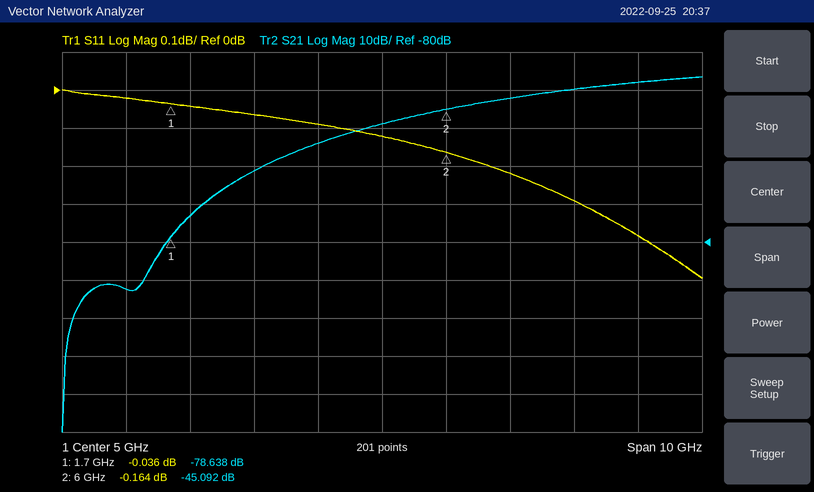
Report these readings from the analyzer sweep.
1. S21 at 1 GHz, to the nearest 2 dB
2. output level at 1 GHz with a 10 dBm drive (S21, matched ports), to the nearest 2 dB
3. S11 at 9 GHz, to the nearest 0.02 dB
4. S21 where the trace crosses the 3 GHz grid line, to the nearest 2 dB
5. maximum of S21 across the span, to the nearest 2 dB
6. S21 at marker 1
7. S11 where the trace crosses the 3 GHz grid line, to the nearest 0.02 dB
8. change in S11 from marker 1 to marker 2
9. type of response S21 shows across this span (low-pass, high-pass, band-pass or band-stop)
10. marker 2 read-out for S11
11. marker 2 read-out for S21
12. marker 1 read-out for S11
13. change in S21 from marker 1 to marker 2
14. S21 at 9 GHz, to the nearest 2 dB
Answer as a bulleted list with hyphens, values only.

- -92 dB
- -82 dBm
- -0.38 dB
- -62 dB
- -36 dB
- -78.638 dB
- -0.06 dB
- -0.128 dB
- high-pass
- -0.164 dB
- -45.092 dB
- -0.036 dB
- 33.546 dB
- -38 dB
